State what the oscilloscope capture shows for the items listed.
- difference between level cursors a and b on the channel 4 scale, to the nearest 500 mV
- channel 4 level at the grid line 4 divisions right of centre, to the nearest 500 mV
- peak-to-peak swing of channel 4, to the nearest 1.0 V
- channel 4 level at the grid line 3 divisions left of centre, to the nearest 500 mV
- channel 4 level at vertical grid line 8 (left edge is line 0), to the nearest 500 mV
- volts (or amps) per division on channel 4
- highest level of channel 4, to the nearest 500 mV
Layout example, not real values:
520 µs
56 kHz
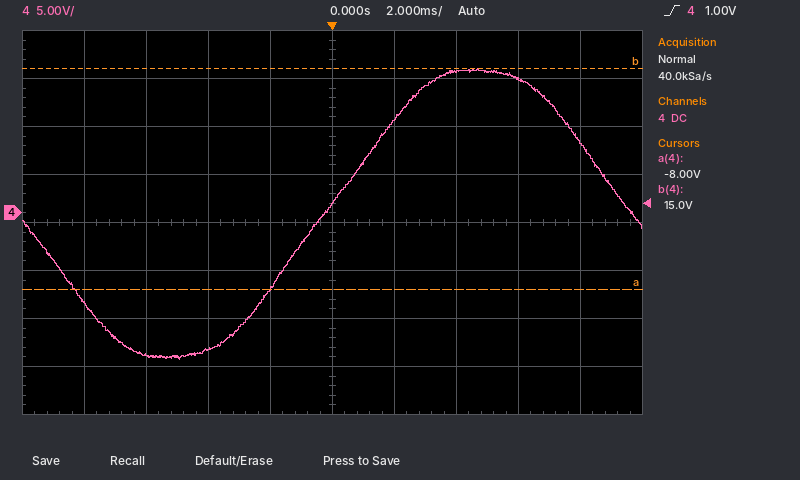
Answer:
23.0 V
7.5 V
30.0 V
-15.0 V
14.0 V
5 V
15.0 V
